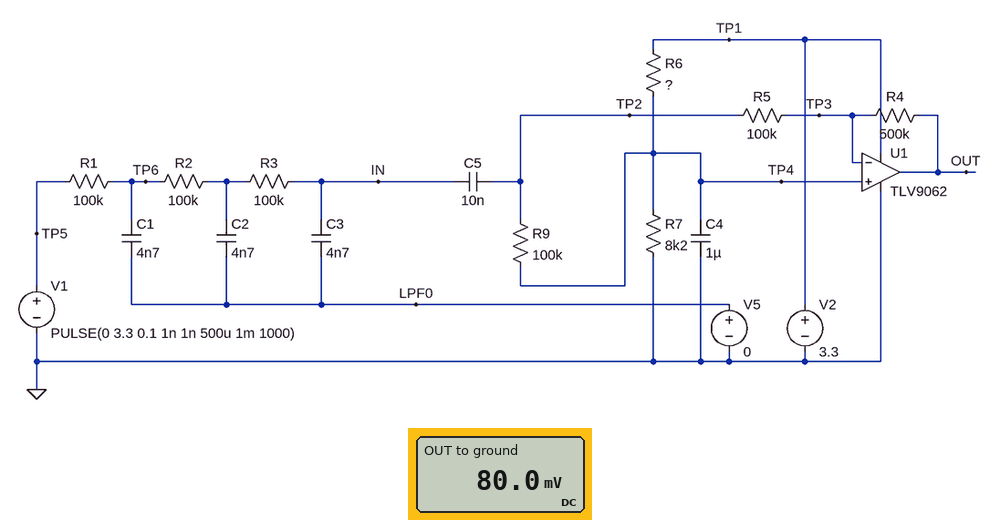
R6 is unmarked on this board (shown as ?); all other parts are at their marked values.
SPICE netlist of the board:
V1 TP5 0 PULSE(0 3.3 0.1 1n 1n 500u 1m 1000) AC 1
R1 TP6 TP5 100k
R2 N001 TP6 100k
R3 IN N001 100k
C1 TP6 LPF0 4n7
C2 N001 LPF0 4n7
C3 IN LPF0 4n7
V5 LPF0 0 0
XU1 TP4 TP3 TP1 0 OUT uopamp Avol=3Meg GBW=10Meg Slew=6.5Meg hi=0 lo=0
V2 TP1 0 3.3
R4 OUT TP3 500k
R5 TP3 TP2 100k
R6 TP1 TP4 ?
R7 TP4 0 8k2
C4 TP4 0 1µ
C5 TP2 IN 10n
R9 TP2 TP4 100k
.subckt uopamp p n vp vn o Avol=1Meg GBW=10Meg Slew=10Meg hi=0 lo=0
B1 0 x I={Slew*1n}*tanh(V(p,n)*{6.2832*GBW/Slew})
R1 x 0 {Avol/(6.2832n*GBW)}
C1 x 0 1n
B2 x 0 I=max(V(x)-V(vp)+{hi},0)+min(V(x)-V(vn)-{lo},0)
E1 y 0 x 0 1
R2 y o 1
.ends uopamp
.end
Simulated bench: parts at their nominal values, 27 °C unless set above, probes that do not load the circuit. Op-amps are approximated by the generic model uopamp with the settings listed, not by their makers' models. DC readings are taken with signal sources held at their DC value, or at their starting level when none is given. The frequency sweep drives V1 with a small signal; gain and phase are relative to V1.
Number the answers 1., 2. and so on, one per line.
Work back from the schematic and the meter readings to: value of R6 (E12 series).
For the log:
1. 330 kΩ
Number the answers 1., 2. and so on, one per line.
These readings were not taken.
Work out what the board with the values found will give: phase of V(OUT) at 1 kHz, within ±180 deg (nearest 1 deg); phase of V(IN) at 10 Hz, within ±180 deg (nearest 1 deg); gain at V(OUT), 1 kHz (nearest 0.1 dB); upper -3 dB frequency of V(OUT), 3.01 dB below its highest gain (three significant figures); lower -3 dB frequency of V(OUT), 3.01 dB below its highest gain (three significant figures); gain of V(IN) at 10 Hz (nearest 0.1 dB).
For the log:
1. 27 deg
2. -20 deg
3. -22.1 dB
4. 333 Hz
5. 24.7 Hz
6. -0.5 dB
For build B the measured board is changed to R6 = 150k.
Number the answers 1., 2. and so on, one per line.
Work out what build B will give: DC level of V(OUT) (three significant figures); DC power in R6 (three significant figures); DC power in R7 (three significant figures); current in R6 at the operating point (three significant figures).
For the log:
1. 171 mV
2. 65.3 µW
3. 3.57 µW
4. 20.9 µA
